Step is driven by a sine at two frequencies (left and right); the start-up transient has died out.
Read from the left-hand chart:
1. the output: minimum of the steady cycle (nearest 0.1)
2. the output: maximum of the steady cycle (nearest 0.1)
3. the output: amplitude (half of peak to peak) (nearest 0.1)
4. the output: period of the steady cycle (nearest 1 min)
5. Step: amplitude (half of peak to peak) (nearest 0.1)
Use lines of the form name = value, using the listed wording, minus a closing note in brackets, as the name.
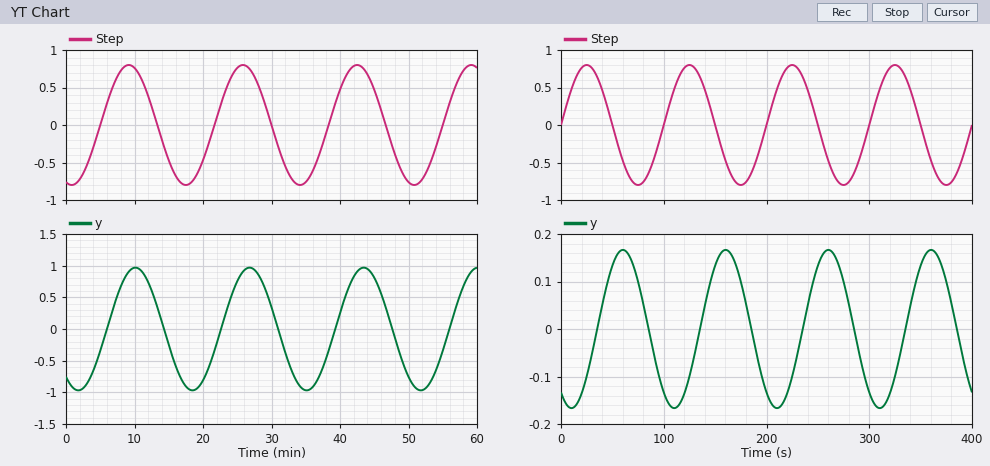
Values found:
the output: minimum of the steady cycle = -1.0
the output: maximum of the steady cycle = 1.0
the output: amplitude (half of peak to peak) = 1.0
the output: period of the steady cycle = 17 min
Step: amplitude (half of peak to peak) = 0.8
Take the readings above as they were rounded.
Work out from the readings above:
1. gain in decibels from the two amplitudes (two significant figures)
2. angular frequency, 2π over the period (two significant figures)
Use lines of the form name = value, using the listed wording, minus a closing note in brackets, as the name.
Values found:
gain in decibels from the two amplitudes = 1.9 dB
angular frequency, 2π over the period = 0.37 rad/min
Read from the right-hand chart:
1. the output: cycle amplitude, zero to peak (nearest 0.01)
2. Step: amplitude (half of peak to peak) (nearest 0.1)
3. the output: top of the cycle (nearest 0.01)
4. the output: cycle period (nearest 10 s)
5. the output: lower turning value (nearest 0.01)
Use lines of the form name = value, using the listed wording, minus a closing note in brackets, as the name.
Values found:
the output: cycle amplitude, zero to peak = 0.17
Step: amplitude (half of peak to peak) = 0.8
the output: top of the cycle = 0.17
the output: cycle period = 100 s
the output: lower turning value = -0.17
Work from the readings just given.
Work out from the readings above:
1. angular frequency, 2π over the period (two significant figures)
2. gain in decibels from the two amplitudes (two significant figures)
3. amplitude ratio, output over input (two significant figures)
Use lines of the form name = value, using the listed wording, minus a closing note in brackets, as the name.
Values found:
angular frequency, 2π over the period = 0.063 rad/s
gain in decibels from the two amplitudes = -13 dB
amplitude ratio, output over input = 0.21
